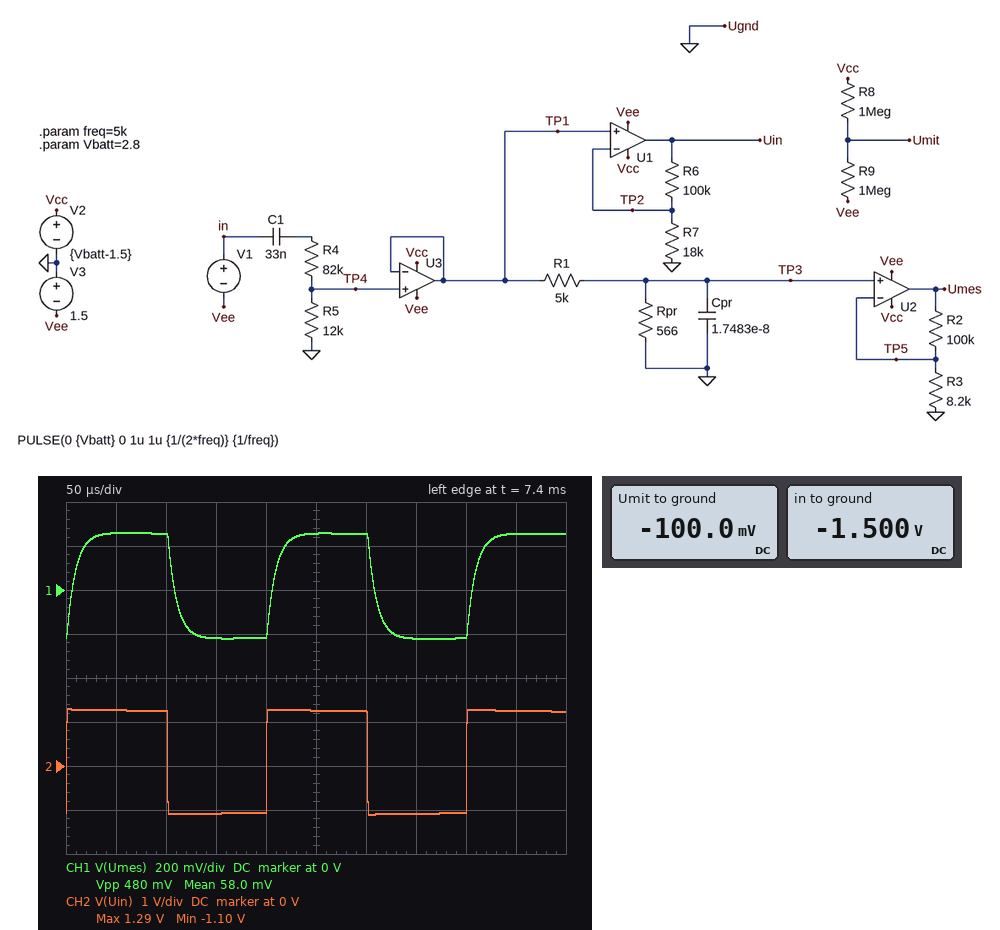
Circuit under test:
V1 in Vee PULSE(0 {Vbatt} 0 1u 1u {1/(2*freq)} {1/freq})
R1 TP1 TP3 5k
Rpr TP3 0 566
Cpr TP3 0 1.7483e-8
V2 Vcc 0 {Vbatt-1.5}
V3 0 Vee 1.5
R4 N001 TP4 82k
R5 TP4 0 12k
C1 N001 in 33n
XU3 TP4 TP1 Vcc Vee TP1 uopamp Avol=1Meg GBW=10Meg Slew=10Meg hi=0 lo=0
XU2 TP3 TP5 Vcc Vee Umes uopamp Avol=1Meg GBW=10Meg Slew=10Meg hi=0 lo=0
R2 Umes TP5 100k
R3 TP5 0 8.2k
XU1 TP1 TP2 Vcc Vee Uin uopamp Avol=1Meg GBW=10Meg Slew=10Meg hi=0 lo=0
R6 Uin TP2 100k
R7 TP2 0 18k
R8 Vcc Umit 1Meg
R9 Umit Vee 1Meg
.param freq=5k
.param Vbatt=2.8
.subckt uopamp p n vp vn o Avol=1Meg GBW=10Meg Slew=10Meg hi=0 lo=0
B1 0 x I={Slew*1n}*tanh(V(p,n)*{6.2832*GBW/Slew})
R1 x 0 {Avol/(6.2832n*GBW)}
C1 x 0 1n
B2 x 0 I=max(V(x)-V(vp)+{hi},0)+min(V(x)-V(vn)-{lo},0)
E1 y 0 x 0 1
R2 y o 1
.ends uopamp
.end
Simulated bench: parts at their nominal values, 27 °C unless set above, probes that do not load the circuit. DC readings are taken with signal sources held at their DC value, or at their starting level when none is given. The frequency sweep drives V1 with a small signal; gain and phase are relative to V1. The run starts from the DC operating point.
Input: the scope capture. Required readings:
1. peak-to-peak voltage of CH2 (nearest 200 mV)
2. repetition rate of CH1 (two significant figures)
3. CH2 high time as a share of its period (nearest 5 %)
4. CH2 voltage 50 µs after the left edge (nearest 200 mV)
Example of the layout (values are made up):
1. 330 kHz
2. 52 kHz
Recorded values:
1. 2.4 V
2. 5.0 kHz
3. 50 %
4. 1.2 V
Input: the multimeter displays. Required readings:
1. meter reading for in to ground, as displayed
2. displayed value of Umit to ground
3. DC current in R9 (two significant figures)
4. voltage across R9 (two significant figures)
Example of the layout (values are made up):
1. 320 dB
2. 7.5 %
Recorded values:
1. -1.500 V
2. -100.0 mV
3. 1.4 µA
4. 1.4 V
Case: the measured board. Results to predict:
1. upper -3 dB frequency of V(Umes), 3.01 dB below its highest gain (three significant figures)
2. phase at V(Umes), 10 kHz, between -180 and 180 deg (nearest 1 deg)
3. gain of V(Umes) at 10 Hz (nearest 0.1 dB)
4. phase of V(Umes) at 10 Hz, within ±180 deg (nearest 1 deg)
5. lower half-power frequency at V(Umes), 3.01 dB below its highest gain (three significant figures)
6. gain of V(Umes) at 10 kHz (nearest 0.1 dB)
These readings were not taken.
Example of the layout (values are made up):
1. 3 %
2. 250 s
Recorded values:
1. 18.0 kHz
2. -30 deg
3. -29.7 dB
4. 79 deg
5. 51.0 Hz
6. -16.5 dB
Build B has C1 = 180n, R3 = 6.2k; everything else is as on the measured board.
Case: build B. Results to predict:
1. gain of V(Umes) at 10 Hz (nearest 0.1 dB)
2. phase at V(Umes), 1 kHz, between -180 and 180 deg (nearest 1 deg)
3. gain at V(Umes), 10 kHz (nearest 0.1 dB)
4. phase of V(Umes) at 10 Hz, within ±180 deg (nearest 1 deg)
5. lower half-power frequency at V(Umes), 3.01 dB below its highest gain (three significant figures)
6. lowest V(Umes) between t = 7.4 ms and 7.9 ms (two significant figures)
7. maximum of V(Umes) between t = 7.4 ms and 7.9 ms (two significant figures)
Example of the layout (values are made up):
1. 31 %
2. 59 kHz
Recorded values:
1. -15.8 dB
2. -3 deg
3. -14.2 dB
4. 43 deg
5. 9.40 Hz
6. -120 mV
7. 510 mV
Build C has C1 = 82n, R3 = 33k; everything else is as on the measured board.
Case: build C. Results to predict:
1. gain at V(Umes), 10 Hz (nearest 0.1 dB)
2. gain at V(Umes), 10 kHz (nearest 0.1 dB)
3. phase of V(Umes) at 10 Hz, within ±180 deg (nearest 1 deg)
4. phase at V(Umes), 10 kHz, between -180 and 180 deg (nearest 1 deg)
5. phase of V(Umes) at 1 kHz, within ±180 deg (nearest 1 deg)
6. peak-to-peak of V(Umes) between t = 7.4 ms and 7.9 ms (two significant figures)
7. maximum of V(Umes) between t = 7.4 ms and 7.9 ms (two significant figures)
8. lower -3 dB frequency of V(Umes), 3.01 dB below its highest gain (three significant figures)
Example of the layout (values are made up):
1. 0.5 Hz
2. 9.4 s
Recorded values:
1. -32.8 dB
2. -26.8 dB
3. 64 deg
4. -29 deg
5. -2 deg
6. 150 mV
7. 100 mV
8. 20.6 Hz
